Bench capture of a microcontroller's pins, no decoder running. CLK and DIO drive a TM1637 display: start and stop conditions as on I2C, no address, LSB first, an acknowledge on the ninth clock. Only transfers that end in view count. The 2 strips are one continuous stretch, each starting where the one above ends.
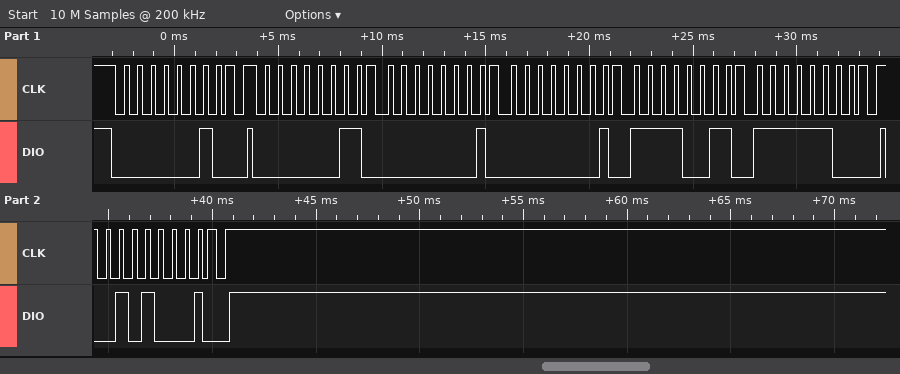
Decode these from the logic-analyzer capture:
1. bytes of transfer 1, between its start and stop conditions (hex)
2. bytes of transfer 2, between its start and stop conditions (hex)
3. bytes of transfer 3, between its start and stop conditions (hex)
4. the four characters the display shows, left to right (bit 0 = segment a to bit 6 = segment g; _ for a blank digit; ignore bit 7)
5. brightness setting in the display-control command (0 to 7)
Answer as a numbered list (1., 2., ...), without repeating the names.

1. 40
2. C0 80 80 CF 3F
3. 8A
4. __30
5. 2
